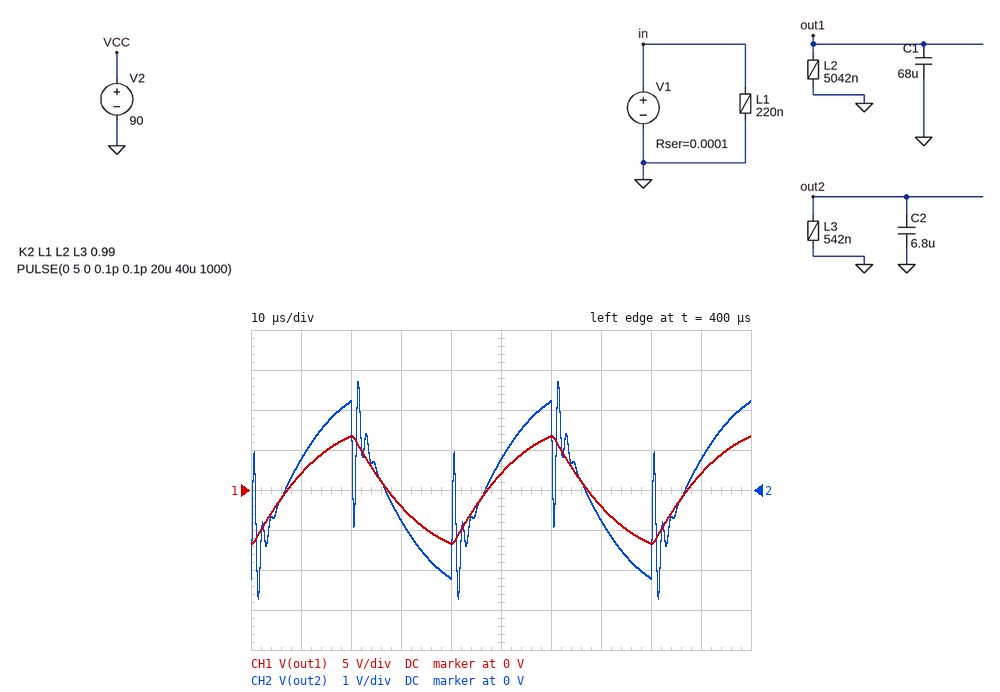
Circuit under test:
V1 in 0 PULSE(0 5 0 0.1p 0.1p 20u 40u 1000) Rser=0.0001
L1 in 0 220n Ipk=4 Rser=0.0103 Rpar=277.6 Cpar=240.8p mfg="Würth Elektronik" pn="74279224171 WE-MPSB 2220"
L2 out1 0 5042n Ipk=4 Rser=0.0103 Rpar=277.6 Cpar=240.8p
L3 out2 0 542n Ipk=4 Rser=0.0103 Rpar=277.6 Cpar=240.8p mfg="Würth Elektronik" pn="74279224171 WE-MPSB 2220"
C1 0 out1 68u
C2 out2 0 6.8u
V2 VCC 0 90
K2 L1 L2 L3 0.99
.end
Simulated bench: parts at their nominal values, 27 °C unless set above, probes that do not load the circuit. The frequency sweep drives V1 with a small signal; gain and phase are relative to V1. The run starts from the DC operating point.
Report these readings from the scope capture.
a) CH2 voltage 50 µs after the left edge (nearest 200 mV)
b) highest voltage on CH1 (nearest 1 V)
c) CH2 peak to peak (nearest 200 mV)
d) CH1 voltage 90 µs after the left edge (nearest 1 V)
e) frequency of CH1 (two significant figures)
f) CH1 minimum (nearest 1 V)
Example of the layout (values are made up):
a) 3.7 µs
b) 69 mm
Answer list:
a) 800 mV
b) 7 V
c) 5.4 V
d) 2 V
e) 25 kHz
f) -7 V
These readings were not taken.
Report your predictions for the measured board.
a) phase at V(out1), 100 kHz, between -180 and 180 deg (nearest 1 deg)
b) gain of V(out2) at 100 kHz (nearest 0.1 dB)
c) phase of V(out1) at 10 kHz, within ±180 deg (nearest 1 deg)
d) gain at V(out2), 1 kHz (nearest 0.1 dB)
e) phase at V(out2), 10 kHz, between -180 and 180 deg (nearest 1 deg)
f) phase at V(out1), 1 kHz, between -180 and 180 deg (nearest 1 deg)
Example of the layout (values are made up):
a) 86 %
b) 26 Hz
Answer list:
a) -99 deg
b) -21.6 dB
c) -18 deg
d) -13.7 dB
e) -15 deg
f) 82 deg
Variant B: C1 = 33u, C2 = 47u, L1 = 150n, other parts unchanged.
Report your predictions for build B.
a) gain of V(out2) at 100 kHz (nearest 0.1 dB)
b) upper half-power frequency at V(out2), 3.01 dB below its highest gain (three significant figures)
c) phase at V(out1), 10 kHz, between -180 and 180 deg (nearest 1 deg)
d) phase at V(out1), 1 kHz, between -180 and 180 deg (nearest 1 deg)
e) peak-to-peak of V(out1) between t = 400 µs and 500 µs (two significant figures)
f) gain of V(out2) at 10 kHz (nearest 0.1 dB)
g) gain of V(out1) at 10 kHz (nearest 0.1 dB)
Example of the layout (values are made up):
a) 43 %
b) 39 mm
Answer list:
a) -19.8 dB
b) 18.7 kHz
c) 14 deg
d) 85 deg
e) 20 V
f) 5.1 dB
g) 14.8 dB
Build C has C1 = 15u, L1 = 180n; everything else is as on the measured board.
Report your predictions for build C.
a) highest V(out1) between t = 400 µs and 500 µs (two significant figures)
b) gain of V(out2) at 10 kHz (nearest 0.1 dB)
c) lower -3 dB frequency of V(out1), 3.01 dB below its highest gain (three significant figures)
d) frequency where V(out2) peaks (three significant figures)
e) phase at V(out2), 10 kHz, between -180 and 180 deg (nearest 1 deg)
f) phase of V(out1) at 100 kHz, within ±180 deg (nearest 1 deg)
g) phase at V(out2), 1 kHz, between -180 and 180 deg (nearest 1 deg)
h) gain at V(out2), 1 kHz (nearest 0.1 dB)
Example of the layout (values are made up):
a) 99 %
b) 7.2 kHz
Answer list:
a) 14 V
b) 3.2 dB
c) 7.65 kHz
d) 17.9 kHz
e) 32 deg
f) -82 deg
g) 84 deg
h) -14.6 dB
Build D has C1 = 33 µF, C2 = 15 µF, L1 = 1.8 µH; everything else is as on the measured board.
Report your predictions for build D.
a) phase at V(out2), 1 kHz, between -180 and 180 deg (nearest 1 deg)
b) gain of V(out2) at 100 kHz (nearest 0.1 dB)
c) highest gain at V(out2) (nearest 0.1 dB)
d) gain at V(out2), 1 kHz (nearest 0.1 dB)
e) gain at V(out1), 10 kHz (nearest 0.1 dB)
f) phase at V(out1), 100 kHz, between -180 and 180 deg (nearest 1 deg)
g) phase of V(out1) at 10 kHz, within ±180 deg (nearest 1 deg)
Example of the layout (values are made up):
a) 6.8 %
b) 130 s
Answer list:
a) 42 deg
b) -11.8 dB
c) -4.5 dB
d) -7.9 dB
e) 4.5 dB
f) -112 deg
g) 0 deg
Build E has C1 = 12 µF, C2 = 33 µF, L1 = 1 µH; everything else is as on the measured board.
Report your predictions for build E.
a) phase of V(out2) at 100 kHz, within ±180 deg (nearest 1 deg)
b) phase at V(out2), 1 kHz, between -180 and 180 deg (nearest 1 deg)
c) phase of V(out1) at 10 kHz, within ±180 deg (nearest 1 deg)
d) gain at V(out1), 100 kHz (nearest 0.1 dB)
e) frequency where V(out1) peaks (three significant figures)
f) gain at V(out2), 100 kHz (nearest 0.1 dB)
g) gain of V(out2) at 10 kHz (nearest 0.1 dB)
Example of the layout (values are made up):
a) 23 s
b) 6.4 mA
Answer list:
a) -56 deg
b) 59 deg
c) 6 deg
d) 9.6 dB
e) 118 kHz
f) -2.0 dB
g) -2.8 dB
